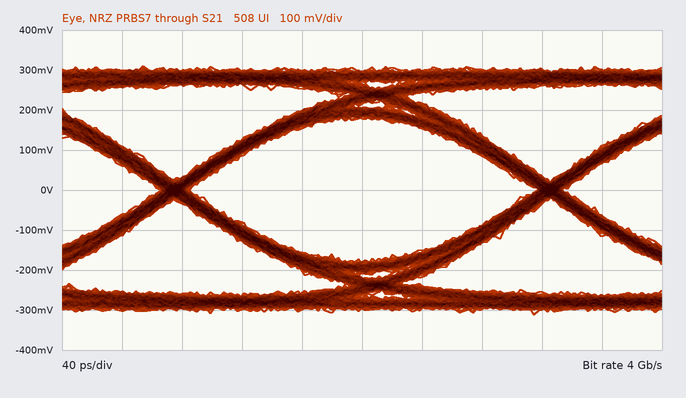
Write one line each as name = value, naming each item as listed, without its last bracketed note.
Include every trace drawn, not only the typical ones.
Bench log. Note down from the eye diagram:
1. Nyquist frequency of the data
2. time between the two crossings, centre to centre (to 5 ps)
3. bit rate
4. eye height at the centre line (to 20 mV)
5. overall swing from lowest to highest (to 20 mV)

Nyquist frequency of the data = 2 GHz
time between the two crossings, centre to centre = 250 ps
bit rate = 4 Gb/s
eye height at the centre line = 360 mV
overall swing from lowest to highest = 620 mV
